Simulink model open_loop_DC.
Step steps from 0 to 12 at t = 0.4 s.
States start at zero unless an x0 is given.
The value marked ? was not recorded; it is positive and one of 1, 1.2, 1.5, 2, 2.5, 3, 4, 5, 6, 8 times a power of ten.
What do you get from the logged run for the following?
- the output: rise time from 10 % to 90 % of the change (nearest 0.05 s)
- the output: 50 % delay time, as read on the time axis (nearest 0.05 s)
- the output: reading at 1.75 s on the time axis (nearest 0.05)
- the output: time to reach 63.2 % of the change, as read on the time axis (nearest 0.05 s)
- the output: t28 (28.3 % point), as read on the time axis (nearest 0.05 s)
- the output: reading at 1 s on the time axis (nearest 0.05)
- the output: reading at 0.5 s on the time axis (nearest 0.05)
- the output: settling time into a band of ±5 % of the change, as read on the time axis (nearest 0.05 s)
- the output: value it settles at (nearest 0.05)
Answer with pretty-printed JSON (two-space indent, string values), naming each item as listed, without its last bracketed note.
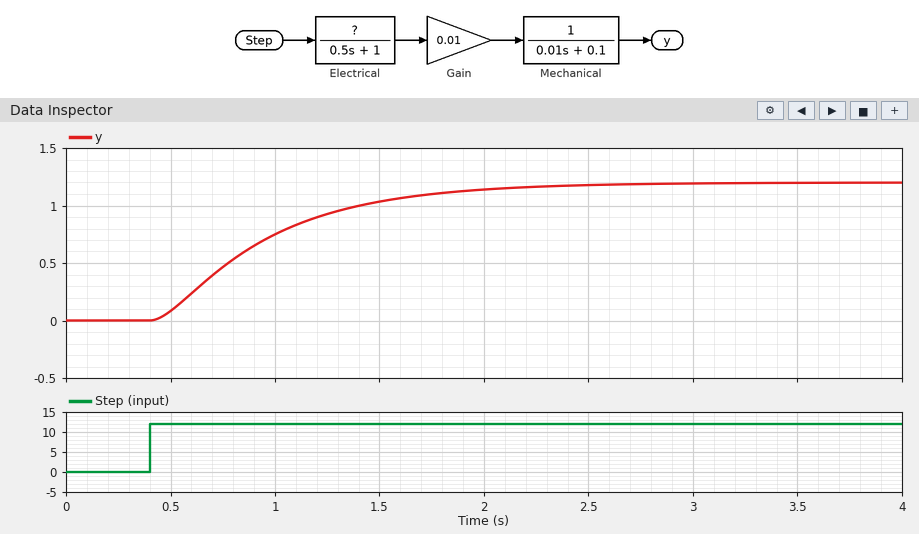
{
  "the output: rise time from 10 % to 90 % of the change": "1.15 s",
  "the output: 50 % delay time, as read on the time axis": "0.85 s",
  "the output: reading at 1.75 s on the time axis": "1.10",
  "the output: time to reach 63.2 % of the change, as read on the time axis": "1.00 s",
  "the output: t28 (28.3 % point), as read on the time axis": "0.65 s",
  "the output: reading at 1 s on the time axis": "0.75",
  "the output: reading at 0.5 s on the time axis": "0.10",
  "the output: settling time into a band of ±5 % of the change, as read on the time axis": "2.00 s",
  "the output: value it settles at": "1.20"
}
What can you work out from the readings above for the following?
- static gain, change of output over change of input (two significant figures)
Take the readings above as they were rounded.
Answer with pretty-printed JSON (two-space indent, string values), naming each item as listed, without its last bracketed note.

{
  "static gain, change of output over change of input": "0.10"
}
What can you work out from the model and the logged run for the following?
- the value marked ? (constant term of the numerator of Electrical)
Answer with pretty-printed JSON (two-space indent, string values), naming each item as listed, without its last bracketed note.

{
  "the value marked ?": "1"
}
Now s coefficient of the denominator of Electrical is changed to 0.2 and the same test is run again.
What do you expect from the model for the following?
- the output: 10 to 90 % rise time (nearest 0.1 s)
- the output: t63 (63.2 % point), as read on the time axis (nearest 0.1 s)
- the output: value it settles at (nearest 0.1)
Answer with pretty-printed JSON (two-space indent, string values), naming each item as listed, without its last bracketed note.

{
  "the output: 10 to 90 % rise time": "0.5 s",
  "the output: t63 (63.2 % point), as read on the time axis": "0.7 s",
  "the output: value it settles at": "1.2"
}
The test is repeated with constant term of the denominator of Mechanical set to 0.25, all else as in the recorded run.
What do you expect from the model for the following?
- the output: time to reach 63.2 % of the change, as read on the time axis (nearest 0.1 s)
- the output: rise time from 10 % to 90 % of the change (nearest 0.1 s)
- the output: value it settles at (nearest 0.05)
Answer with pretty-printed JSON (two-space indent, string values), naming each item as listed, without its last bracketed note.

{
  "the output: time to reach 63.2 % of the change, as read on the time axis": "0.9 s",
  "the output: rise time from 10 % to 90 % of the change": "1.1 s",
  "the output: value it settles at": "0.50"
}
